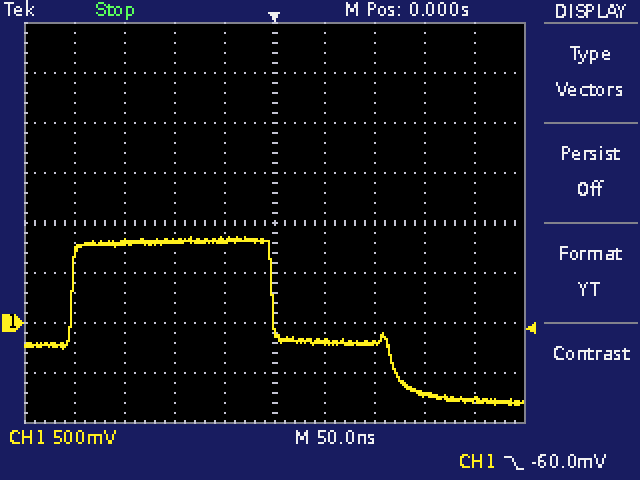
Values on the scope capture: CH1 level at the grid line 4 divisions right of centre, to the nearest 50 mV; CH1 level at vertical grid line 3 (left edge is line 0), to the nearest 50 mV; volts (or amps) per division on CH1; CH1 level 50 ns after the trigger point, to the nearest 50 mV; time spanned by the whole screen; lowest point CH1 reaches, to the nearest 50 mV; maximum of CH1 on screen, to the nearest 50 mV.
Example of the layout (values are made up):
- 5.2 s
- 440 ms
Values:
- -750 mV
- 800 mV
- 500 mV
- -200 mV
- 500 ns
- -800 mV
- 850 mV
